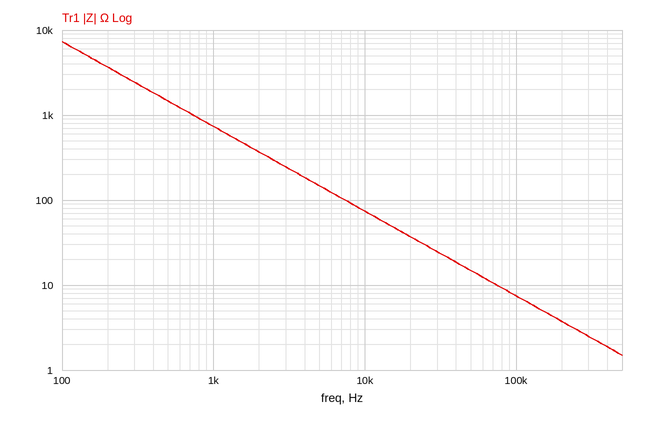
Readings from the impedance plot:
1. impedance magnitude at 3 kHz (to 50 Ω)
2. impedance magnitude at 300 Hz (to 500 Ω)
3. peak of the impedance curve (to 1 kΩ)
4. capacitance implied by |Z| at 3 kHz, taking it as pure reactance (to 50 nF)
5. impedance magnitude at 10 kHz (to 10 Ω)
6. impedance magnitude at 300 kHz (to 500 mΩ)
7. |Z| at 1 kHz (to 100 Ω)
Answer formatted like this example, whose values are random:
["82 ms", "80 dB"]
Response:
["250 Ω", "2.5 kΩ", "7 kΩ", "200 nF", "70 Ω", "2.5 Ω", "700 Ω"]
